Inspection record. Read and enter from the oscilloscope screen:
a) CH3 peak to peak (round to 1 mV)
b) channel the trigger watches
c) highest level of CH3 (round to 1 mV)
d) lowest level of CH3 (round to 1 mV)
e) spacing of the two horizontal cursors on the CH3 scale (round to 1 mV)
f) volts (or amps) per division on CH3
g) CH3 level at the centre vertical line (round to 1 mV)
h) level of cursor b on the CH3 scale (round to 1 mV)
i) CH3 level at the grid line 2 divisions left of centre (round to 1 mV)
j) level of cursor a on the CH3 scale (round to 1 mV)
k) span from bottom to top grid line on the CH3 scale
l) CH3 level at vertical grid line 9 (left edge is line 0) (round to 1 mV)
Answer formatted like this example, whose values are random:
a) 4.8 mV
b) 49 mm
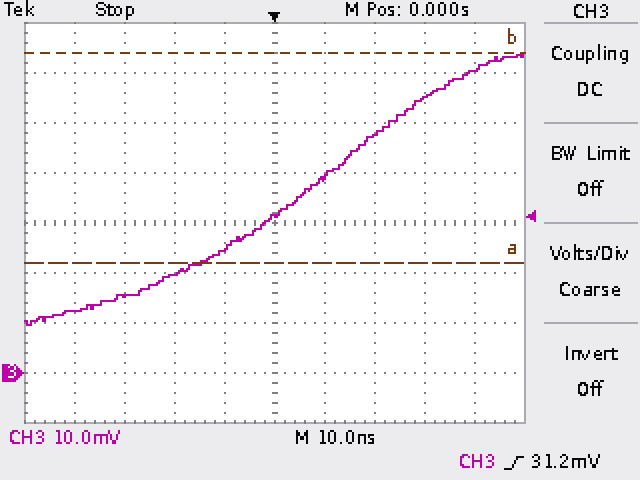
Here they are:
a) 54 mV
b) CH3
c) 64 mV
d) 10 mV
e) 42 mV
f) 10 mV
g) 31 mV
h) 64 mV
i) 20 mV
j) 22 mV
k) 80 mV
l) 61 mV
